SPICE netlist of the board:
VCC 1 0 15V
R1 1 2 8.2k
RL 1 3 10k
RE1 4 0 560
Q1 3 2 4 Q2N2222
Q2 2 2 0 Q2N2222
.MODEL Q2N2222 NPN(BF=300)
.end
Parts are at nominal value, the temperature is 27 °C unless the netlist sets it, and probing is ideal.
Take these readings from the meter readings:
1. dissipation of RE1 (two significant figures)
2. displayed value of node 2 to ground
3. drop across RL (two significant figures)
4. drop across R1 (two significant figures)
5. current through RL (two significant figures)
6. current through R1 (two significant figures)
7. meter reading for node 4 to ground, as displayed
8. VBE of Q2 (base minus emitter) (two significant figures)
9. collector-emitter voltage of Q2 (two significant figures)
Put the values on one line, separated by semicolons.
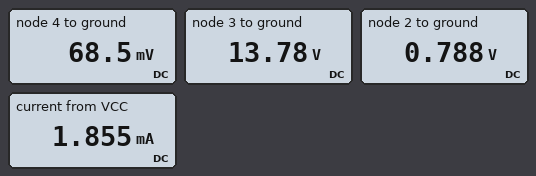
8.4 µW; 0.788 V; 1.2 V; 14 V; 120 µA; 1.7 mA; 68.5 mV; 790 mV; 790 mV
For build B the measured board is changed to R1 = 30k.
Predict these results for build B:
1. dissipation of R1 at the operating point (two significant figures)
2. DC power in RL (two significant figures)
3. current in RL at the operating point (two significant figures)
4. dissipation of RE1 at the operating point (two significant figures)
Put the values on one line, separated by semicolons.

6.8 mW; 66 µW; 81 µA; 3.7 µW
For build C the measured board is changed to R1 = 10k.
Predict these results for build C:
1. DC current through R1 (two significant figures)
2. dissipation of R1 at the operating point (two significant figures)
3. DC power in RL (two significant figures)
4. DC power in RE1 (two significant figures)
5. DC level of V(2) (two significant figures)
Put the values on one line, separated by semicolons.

1.4 mA; 20 mW; 130 µW; 7.5 µW; 780 mV
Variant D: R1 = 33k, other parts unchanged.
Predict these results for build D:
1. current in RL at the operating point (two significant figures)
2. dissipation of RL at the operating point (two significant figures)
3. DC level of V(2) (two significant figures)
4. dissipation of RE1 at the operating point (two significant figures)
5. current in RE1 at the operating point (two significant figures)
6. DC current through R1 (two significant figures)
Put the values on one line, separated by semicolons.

78 µA; 61 µW; 750 mV; 3.5 µW; 79 µA; 430 µA
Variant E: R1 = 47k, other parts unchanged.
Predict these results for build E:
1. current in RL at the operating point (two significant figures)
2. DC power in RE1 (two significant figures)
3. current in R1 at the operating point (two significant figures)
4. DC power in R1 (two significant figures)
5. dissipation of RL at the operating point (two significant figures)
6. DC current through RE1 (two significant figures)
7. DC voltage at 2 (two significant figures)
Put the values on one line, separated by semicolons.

68 µA; 2.6 µW; 300 µA; 4.3 mW; 47 µW; 69 µA; 740 mV
